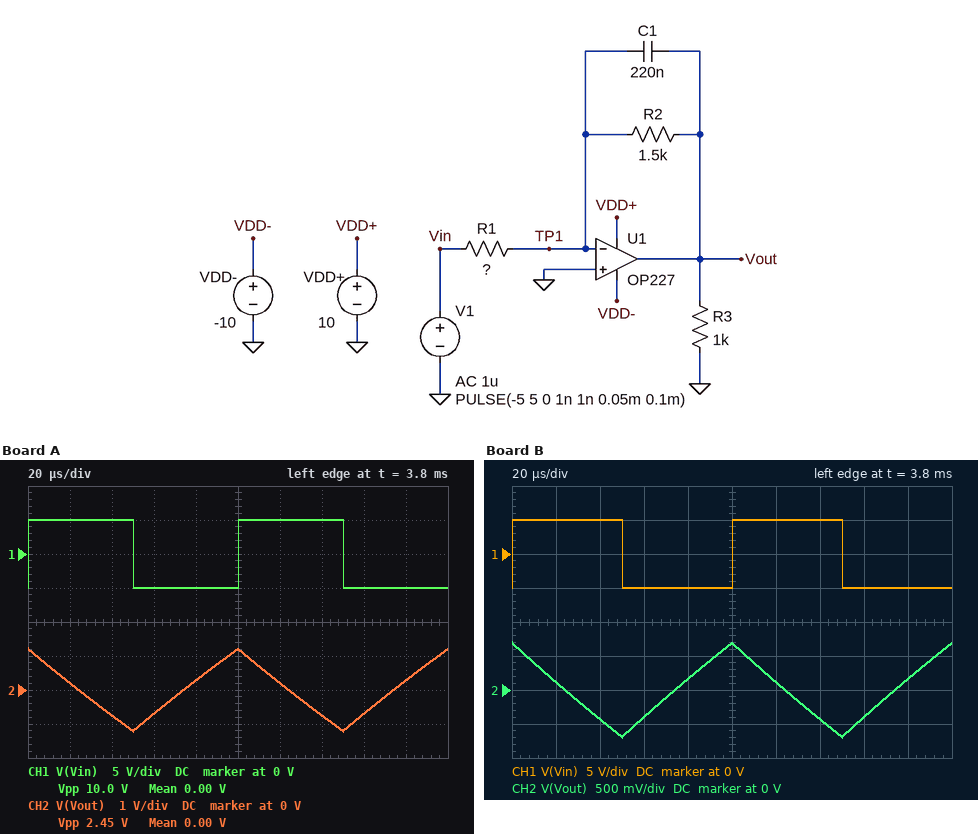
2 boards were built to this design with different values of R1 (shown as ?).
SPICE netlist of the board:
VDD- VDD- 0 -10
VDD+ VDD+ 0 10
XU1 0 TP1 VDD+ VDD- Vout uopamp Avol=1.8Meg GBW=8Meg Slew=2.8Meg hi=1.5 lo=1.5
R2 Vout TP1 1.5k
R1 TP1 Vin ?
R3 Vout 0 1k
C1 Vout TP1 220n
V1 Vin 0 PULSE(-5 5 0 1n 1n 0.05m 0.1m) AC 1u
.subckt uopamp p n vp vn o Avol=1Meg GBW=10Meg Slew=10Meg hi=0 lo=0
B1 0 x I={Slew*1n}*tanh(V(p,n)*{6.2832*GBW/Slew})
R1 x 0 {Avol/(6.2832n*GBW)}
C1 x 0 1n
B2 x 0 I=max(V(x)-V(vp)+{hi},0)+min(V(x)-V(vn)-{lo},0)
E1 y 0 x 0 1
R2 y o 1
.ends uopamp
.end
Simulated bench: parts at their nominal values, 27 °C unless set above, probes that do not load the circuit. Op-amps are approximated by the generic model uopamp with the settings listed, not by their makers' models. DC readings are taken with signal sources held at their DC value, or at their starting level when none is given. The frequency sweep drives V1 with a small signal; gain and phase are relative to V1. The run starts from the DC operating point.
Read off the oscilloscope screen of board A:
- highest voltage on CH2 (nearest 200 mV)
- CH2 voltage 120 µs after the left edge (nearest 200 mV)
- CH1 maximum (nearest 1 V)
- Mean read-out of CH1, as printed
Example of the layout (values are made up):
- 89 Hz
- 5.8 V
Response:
- 1.2 V
- 200 mV
- 5 V
- 0.00 V
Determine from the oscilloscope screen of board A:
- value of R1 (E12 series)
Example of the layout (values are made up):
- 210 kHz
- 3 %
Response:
- 470 Ω
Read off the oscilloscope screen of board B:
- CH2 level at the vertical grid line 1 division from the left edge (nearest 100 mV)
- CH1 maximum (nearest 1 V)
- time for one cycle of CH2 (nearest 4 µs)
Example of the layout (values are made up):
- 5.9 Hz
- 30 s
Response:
- 100 mV
- 5 V
- 100 µs
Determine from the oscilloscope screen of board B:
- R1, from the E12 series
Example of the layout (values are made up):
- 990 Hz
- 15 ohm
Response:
- 820 Ω
